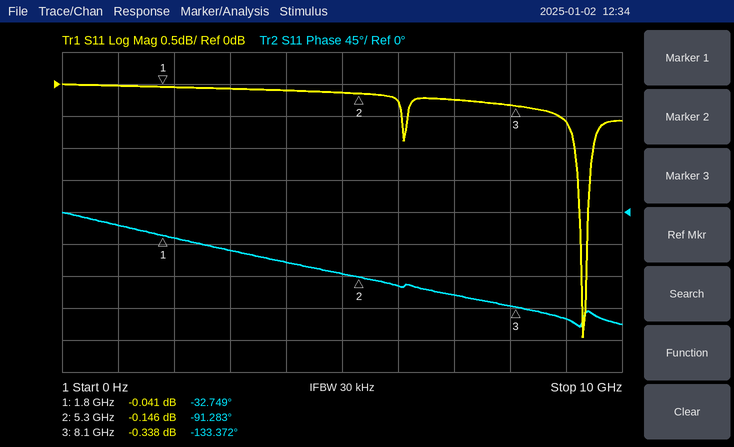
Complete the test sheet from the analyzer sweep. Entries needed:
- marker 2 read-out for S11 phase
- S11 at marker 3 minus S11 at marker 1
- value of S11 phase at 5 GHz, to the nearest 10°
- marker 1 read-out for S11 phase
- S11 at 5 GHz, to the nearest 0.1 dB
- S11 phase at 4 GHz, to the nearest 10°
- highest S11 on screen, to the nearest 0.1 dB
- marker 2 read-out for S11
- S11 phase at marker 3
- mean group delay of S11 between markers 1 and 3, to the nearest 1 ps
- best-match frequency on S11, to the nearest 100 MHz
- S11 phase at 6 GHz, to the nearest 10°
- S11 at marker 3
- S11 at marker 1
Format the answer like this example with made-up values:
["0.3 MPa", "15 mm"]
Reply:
["-91.283°", "-0.297 dB", "-90°", "-32.749°", "-0.1 dB", "-70°", "0.0 dB", "-0.146 dB", "-133.372°", "44 ps", "9.3 GHz", "-100°", "-0.338 dB", "-0.041 dB"]
